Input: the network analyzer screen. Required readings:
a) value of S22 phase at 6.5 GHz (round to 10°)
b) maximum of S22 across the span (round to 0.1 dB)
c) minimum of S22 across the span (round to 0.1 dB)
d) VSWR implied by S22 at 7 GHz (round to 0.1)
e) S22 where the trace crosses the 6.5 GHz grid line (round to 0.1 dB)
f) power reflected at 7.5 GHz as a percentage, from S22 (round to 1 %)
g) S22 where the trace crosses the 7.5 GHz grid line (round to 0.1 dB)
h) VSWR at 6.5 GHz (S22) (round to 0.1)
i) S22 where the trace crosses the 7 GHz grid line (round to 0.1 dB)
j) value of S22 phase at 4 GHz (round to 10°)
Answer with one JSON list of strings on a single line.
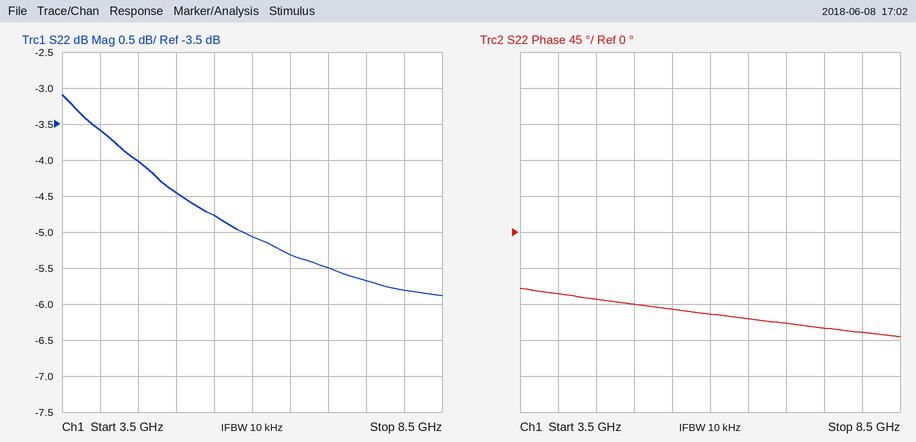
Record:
["-110°", "-3.1 dB", "-5.9 dB", "3.3", "-5.3 dB", "27 %", "-5.7 dB", "3.4", "-5.5 dB", "-80°"]
